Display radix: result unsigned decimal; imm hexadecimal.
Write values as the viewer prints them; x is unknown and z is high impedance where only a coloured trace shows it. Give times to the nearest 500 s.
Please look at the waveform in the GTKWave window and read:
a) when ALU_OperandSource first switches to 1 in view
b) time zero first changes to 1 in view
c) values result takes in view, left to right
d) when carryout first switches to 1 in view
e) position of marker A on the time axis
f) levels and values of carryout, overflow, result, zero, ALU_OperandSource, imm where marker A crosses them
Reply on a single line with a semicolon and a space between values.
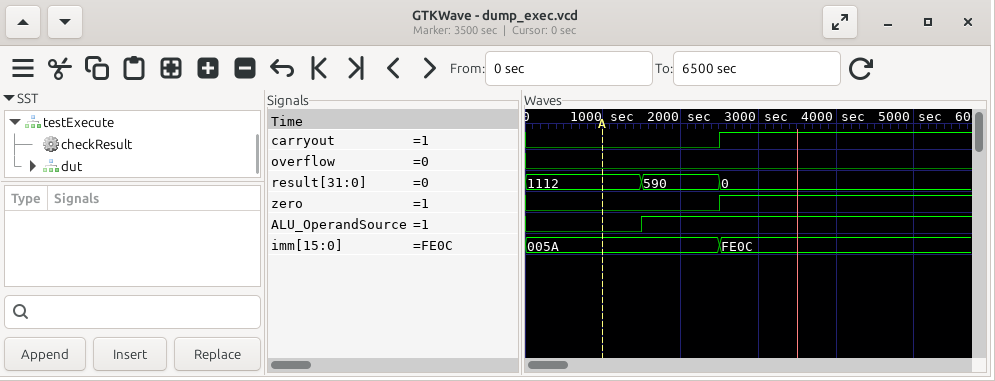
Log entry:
1500 s; 2500 s; 1112, 590, 0; 2500 s; 1000 s; carryout=0, overflow=0, result=1112, zero=0, ALU_OperandSource=0, imm=005A
